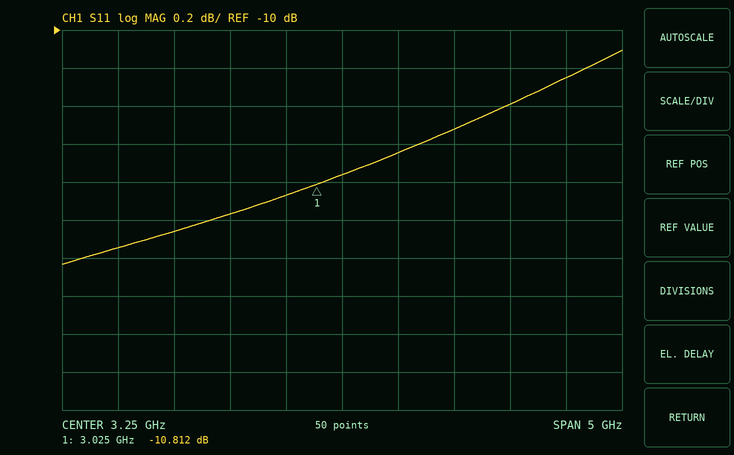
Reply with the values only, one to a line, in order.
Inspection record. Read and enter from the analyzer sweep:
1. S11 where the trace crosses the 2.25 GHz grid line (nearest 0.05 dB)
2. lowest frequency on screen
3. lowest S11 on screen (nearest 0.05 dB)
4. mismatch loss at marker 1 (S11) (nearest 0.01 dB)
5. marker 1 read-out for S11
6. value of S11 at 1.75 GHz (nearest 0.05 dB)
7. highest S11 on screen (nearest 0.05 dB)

-10.95 dB
750 MHz
-11.25 dB
0.38 dB
-10.812 dB
-11.05 dB
-10.10 dB
